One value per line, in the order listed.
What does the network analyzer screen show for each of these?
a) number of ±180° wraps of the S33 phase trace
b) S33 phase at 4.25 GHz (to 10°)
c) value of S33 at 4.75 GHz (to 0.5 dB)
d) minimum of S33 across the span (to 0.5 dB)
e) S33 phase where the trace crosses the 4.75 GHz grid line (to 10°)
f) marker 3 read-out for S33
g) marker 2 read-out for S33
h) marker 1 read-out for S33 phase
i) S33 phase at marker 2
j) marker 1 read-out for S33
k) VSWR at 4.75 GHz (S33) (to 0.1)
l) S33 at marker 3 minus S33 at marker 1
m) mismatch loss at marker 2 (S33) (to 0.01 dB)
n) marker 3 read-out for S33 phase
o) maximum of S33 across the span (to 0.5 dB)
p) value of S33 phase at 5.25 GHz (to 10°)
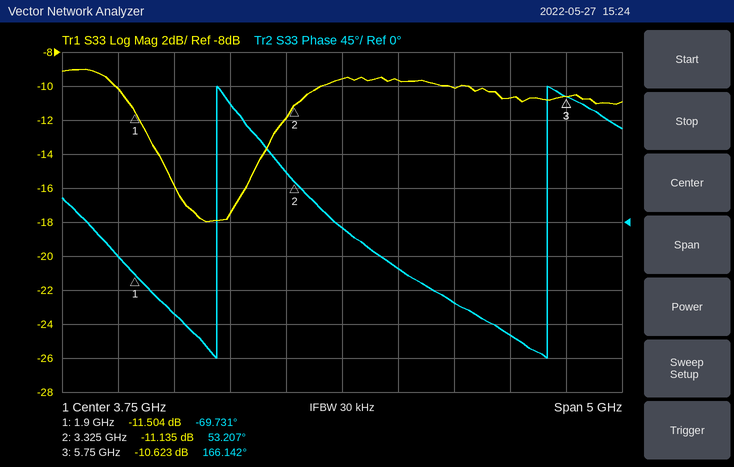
2
-60°
-10.0 dB
-18.0 dB
-110°
-10.623 dB
-11.135 dB
-69.731°
53.207°
-11.504 dB
1.9
0.881 dB
0.35 dB
166.142°
-9.0 dB
-150°
